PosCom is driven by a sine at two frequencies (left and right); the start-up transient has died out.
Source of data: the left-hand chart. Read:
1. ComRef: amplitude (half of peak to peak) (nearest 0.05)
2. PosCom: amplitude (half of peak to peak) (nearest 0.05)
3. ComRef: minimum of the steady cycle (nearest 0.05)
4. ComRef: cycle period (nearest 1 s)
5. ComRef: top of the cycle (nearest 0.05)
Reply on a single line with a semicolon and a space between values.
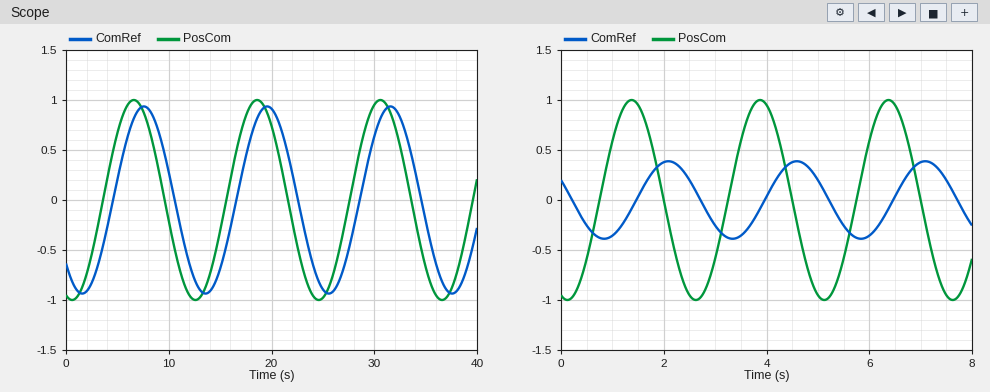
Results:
0.95; 1.00; -0.95; 12 s; 0.95
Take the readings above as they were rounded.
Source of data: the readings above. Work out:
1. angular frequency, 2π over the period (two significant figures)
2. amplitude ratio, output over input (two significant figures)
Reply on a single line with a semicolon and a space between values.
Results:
0.52 rad/s; 0.95
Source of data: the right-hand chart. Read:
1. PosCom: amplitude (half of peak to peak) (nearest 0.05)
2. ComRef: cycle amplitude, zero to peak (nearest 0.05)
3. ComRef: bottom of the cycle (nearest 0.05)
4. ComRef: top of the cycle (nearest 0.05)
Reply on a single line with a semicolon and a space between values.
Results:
1.00; 0.40; -0.40; 0.40
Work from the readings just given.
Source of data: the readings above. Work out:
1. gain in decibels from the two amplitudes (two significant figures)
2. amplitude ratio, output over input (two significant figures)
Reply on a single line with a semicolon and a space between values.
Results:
-8.0 dB; 0.40
